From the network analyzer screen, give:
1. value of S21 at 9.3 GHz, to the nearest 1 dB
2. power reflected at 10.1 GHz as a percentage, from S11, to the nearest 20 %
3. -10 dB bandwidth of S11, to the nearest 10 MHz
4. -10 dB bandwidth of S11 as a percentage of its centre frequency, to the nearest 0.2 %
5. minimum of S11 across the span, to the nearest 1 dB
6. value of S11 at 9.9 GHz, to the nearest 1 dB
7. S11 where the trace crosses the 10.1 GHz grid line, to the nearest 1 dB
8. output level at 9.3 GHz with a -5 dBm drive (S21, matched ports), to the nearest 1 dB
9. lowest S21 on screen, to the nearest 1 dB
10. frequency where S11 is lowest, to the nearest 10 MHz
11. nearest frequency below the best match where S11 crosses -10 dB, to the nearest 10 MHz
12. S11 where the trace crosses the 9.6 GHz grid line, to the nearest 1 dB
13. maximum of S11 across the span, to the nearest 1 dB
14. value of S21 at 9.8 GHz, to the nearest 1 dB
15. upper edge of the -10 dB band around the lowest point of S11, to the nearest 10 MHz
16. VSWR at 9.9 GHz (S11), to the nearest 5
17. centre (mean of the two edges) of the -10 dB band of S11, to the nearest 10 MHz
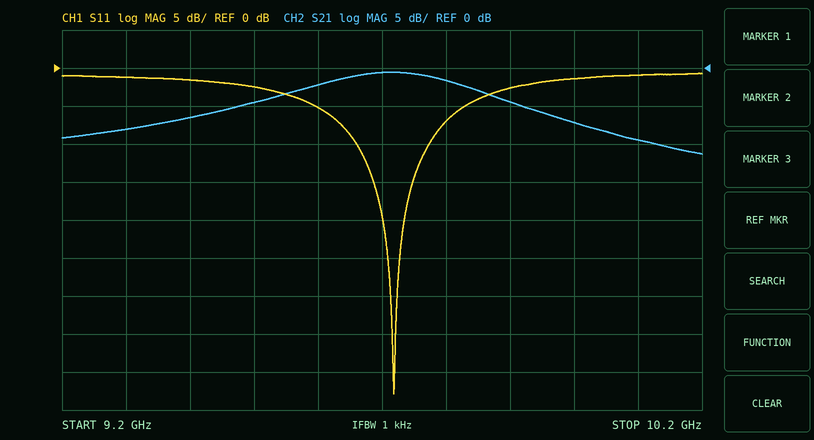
-8 dB
80 %
110 MHz
1.2 %
-43 dB
-3 dB
-1 dB
-13 dBm
-11 dB
9.72 GHz
9.66 GHz
-5 dB
-1 dB
-2 dB
9.77 GHz
5
9.72 GHz
